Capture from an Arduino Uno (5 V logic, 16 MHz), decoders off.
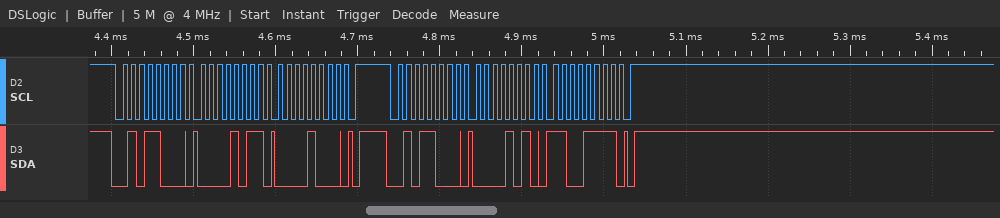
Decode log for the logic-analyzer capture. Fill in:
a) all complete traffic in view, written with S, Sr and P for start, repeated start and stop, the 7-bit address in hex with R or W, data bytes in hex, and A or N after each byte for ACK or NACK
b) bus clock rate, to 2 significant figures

S 2CW A 0B A 08 A P S 2CW A 0A A CF A P
100 kHz
